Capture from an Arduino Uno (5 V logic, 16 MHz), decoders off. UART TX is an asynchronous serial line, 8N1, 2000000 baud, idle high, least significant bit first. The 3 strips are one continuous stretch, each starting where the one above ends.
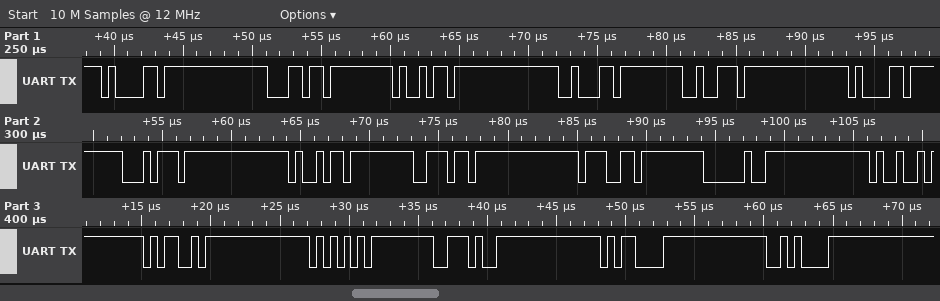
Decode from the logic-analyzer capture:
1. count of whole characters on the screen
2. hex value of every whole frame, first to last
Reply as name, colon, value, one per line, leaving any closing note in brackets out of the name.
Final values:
count of whole characters on the screen: 17
hex value of every whole frame, first to last: 0x61 0x6C 0x69 0x62 0x72 0x61 0x74 0x69 0x6E 0x67 0x20 0x49 0x4D 0x55 0x2E 0x0D 0x0A
